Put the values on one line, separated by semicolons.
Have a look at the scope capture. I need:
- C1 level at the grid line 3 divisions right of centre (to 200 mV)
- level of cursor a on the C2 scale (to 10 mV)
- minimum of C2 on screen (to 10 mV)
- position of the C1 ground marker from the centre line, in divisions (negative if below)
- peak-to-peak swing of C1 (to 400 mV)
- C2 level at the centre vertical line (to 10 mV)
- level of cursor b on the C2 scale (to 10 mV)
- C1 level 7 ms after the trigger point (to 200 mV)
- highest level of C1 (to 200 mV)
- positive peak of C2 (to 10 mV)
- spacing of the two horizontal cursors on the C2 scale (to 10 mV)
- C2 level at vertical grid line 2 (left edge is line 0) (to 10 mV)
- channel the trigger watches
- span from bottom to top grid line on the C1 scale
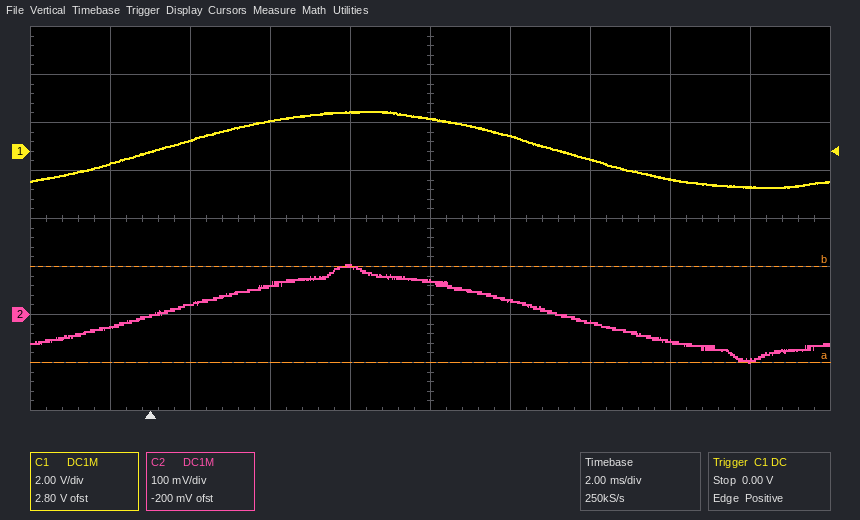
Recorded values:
-1.2 V; -100 mV; -100 mV; +1.4 div; 3.2 V; 70 mV; 100 mV; 1.4 V; 1.6 V; 100 mV; 200 mV; 20 mV; C1; 16 V
